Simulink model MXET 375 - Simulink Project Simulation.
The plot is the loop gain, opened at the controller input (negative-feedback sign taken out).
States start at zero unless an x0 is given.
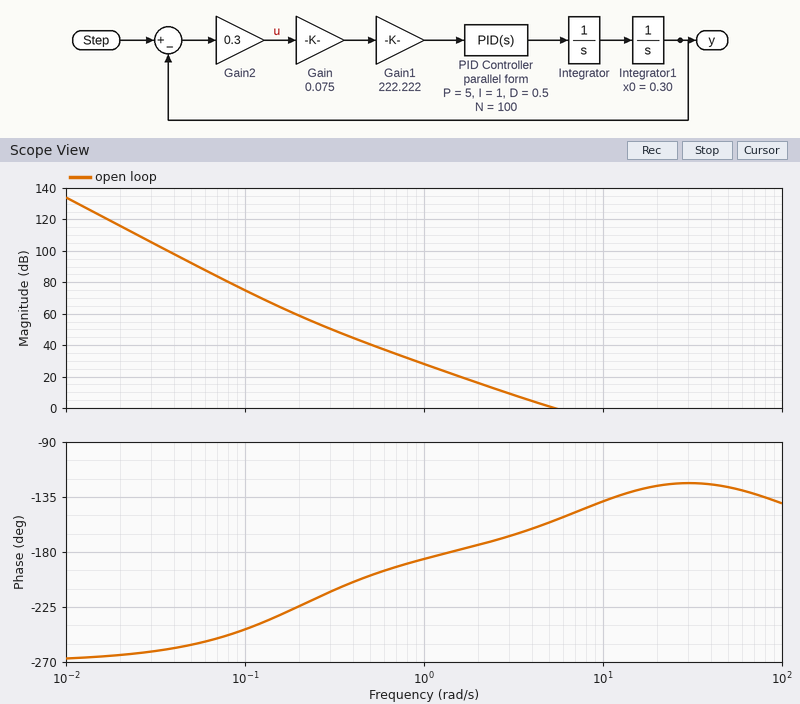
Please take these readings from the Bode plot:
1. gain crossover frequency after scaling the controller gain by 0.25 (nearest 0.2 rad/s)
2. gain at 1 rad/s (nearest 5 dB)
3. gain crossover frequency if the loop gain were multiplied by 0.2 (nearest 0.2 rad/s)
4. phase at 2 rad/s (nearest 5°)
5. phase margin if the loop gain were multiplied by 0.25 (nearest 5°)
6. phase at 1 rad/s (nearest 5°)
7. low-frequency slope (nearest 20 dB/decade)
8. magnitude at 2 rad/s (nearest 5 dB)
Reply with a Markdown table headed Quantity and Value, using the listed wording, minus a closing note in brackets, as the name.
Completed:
| Quantity | Value |
|---|---|
| gain crossover frequency after scaling the controller gain by 0.25 | 2.6 rad/s |
| gain at 1 rad/s | 30 dB |
| gain crossover frequency if the loop gain were multiplied by 0.2 | 2.2 rad/s |
| phase at 2 rad/s | -175° |
| phase margin if the loop gain were multiplied by 0.25 | 10° |
| phase at 1 rad/s | -185° |
| low-frequency slope | -60 dB/decade |
| magnitude at 2 rad/s | 15 dB |
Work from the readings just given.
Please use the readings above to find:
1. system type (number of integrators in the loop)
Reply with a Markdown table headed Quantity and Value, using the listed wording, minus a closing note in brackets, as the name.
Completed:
| Quantity | Value |
|---|---|
| system type | 3 |
